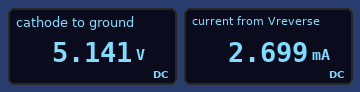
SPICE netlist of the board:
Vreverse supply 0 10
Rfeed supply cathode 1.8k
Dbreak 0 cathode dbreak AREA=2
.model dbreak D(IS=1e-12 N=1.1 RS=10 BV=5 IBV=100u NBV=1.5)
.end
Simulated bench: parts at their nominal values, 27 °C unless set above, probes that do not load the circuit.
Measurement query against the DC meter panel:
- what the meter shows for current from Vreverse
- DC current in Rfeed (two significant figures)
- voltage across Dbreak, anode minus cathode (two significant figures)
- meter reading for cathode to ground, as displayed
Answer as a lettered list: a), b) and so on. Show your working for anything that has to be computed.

a) 2.699 mA
b) (10 V - 5.141 V) / 1.8 kΩ = 2.7 mA
c) 0 V - 5.141 V = -5.1 V
d) 5.141 V
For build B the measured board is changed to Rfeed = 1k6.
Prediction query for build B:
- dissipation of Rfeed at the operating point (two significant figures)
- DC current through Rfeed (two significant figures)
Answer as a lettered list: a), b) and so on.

a) 15 mW
b) 3.0 mA
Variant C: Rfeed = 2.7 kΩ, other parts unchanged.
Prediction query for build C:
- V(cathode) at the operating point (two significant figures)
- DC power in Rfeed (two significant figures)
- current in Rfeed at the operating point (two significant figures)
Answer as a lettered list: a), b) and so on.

a) 5.1 V
b) 8.8 mW
c) 1.8 mA
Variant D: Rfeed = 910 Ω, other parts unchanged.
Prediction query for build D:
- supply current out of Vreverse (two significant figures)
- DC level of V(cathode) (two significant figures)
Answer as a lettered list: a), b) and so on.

a) 5.3 mA
b) 5.2 V
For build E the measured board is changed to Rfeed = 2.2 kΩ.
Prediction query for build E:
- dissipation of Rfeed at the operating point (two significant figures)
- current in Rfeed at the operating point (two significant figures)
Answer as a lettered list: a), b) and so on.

a) 11 mW
b) 2.2 mA
